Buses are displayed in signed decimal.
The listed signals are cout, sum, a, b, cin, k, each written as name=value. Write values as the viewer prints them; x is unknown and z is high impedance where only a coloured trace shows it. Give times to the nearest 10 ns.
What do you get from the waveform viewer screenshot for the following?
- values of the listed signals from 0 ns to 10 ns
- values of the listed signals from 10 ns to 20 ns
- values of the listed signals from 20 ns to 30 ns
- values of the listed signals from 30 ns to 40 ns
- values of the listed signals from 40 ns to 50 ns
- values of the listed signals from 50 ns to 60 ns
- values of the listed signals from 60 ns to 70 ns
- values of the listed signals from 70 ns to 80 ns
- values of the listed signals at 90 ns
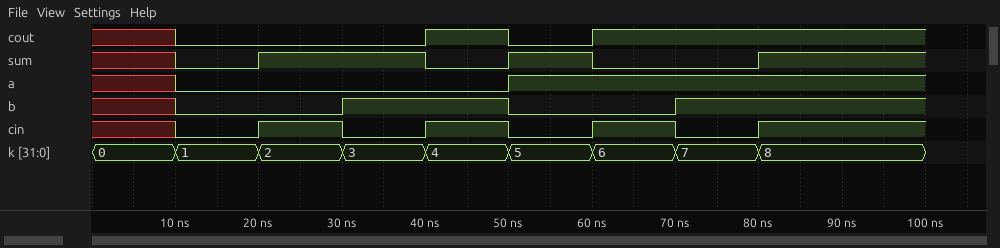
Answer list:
cout=x, sum=x, a=x, b=x, cin=x, k=0
cout=0, sum=0, a=0, b=0, cin=0, k=1
cout=0, sum=1, a=0, b=0, cin=1, k=2
cout=0, sum=1, a=0, b=1, cin=0, k=3
cout=1, sum=0, a=0, b=1, cin=1, k=4
cout=0, sum=1, a=1, b=0, cin=0, k=5
cout=1, sum=0, a=1, b=0, cin=1, k=6
cout=1, sum=0, a=1, b=1, cin=0, k=7
cout=1, sum=1, a=1, b=1, cin=1, k=8
